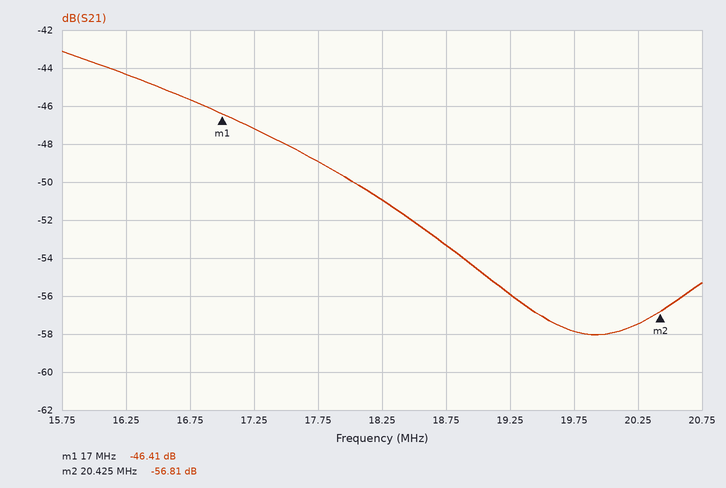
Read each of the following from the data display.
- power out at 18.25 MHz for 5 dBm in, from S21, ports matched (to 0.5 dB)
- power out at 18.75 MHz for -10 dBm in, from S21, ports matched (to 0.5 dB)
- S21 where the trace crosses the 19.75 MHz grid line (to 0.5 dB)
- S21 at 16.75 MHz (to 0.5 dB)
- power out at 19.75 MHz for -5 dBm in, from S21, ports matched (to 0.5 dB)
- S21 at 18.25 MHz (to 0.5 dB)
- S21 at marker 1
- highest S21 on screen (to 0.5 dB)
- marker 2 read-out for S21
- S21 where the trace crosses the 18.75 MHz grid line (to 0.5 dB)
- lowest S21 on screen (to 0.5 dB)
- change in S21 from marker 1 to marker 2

-46.0 dBm
-63.5 dBm
-58.0 dB
-45.5 dB
-63.0 dBm
-51.0 dB
-46.41 dB
-43.0 dB
-56.81 dB
-53.5 dB
-58.0 dB
-10.40 dB
